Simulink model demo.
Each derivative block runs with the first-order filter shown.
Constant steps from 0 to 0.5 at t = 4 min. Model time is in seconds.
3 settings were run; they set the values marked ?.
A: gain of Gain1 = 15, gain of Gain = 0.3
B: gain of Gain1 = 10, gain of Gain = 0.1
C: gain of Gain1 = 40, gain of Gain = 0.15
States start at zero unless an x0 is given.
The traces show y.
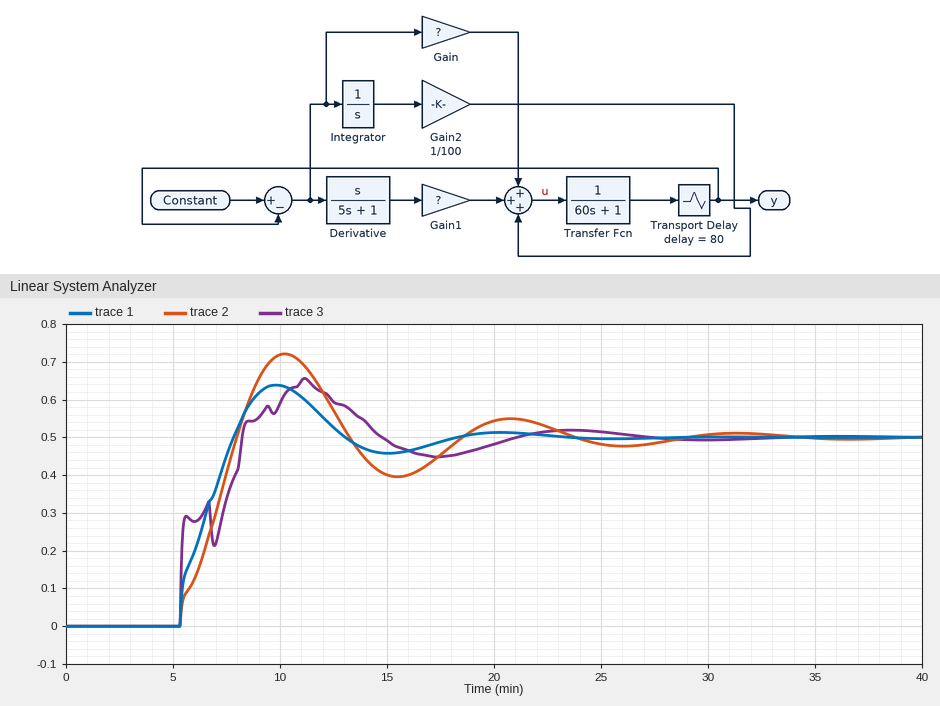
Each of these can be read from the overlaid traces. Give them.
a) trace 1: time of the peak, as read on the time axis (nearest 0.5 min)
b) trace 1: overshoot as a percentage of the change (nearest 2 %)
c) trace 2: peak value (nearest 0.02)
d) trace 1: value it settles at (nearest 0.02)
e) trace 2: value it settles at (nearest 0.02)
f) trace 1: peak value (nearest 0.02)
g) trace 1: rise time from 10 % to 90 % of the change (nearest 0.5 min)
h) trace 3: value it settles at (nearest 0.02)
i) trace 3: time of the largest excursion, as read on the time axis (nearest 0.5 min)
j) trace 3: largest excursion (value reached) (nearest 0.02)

10.0 min
28 %
0.72
0.50
0.50
0.64
2.0 min
0.50
11.0 min
0.66
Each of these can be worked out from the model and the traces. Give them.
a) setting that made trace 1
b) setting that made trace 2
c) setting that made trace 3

A
B
C
